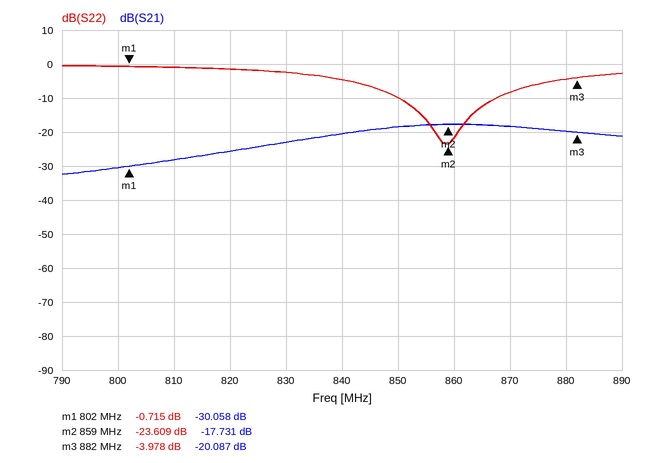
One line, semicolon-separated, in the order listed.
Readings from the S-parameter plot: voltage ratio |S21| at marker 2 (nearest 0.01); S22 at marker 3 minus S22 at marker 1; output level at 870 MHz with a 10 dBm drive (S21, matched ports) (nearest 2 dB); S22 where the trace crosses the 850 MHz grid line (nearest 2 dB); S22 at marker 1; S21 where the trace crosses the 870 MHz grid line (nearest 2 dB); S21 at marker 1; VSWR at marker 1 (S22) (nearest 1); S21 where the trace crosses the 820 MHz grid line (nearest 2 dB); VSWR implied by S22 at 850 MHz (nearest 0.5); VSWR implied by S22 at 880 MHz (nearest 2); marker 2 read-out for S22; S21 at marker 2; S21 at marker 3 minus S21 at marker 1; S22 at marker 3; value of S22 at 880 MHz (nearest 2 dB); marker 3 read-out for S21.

0.13; -3.263 dB; -8 dBm; -10 dB; -0.715 dB; -18 dB; -30.058 dB; 24; -26 dB; 2.0; 4; -23.609 dB; -17.731 dB; 9.971 dB; -3.978 dB; -4 dB; -20.087 dB
